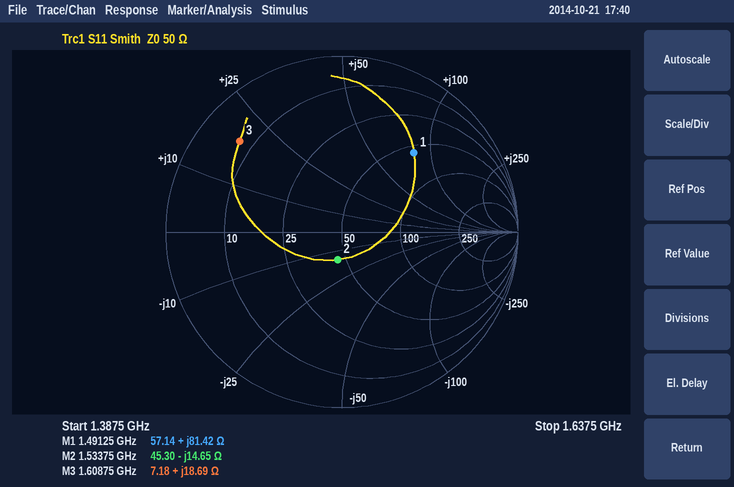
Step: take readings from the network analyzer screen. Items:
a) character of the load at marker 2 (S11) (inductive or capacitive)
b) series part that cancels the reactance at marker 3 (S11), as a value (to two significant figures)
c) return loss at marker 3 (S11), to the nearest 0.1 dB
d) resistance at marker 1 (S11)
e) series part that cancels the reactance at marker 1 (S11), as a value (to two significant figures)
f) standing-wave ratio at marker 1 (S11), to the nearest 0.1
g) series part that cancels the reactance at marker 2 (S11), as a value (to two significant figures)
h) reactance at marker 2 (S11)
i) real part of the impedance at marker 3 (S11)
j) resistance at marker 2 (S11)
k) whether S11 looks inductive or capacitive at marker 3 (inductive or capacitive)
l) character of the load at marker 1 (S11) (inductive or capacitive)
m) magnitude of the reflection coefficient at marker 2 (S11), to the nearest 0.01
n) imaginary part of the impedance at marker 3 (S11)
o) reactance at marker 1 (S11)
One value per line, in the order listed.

capacitive
5.3 pF
2.2 dB
57.14 Ω
1.3 pF
4.1
1.5 nH
-14.65 Ω
7.18 Ω
45.30 Ω
inductive
inductive
0.16
+18.69 Ω
+81.42 Ω
